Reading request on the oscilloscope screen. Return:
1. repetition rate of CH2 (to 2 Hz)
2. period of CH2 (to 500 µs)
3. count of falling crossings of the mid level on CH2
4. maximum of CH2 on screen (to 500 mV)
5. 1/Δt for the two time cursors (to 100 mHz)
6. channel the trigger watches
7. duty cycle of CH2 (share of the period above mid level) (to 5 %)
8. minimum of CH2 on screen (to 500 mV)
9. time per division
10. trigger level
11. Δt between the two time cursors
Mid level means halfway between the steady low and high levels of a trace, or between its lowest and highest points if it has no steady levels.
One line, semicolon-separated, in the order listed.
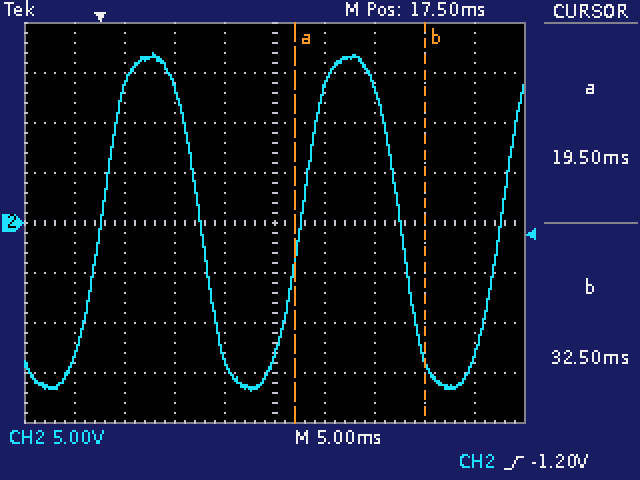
50 Hz; 20.0 ms; 2; 17.0 V; 76.9 Hz; CH2; 50 %; -17.0 V; 5 ms; -1.20 V; 13.0 ms
